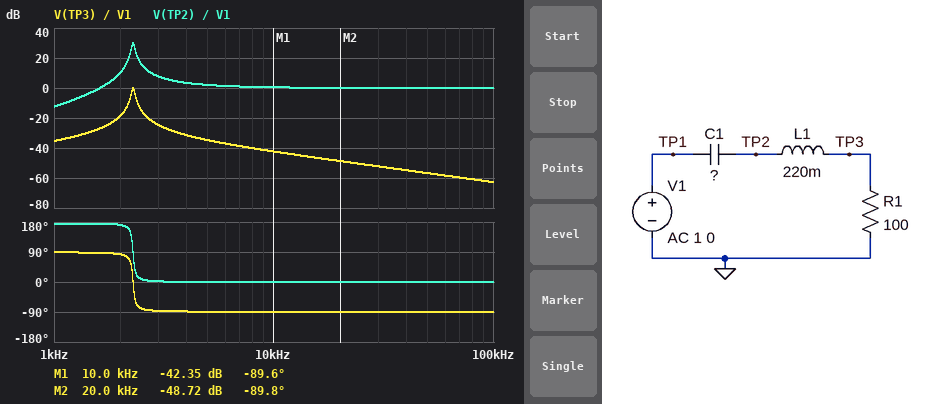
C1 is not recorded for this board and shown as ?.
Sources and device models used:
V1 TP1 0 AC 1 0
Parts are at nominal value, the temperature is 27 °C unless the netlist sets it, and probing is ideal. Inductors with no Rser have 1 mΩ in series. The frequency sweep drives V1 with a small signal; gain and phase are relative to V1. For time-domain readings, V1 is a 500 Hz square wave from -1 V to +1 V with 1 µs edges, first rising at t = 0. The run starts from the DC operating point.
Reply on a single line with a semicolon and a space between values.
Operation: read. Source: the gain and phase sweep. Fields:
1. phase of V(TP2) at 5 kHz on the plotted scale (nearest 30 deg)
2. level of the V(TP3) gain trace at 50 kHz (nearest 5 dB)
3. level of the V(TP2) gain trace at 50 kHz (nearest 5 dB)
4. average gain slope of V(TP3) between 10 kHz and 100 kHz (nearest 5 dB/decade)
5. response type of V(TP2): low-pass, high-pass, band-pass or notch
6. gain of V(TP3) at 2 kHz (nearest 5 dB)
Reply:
0 deg; -55 dB; 0 dB; -20 dB/decade; high-pass; -20 dB
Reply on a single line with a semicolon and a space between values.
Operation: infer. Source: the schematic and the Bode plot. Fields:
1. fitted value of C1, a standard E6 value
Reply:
22 nF
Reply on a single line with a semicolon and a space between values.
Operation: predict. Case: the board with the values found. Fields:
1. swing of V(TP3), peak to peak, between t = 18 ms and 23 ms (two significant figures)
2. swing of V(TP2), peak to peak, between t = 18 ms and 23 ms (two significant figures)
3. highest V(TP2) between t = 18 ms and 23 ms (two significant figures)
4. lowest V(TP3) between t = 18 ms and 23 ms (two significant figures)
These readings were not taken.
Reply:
110 mV; 3.5 V; 1.8 V; -54 mV
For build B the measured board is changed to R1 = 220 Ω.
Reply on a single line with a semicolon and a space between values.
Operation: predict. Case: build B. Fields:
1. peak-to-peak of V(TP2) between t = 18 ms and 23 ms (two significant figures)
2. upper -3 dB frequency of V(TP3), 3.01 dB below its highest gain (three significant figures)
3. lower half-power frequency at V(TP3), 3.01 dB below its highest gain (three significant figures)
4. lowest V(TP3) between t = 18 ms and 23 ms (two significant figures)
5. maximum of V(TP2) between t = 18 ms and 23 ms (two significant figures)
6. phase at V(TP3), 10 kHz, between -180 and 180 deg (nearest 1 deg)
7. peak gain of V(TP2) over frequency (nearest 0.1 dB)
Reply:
3.7 V; 2.37 kHz; 2.21 kHz; -120 mV; 1.9 V; -89 deg; 23.2 dB
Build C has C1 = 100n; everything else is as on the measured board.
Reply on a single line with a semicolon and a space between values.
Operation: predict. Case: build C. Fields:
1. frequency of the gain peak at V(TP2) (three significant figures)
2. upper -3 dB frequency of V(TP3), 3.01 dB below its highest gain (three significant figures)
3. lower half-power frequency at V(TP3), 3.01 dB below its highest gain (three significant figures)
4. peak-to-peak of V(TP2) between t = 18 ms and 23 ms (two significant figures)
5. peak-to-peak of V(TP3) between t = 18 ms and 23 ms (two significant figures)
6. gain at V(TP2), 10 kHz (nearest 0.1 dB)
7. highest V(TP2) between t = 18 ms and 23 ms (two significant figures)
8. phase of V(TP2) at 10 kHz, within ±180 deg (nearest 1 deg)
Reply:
1.07 kHz; 1.11 kHz; 1.04 kHz; 2.3 V; 150 mV; 0.1 dB; 1.1 V; 0 deg
